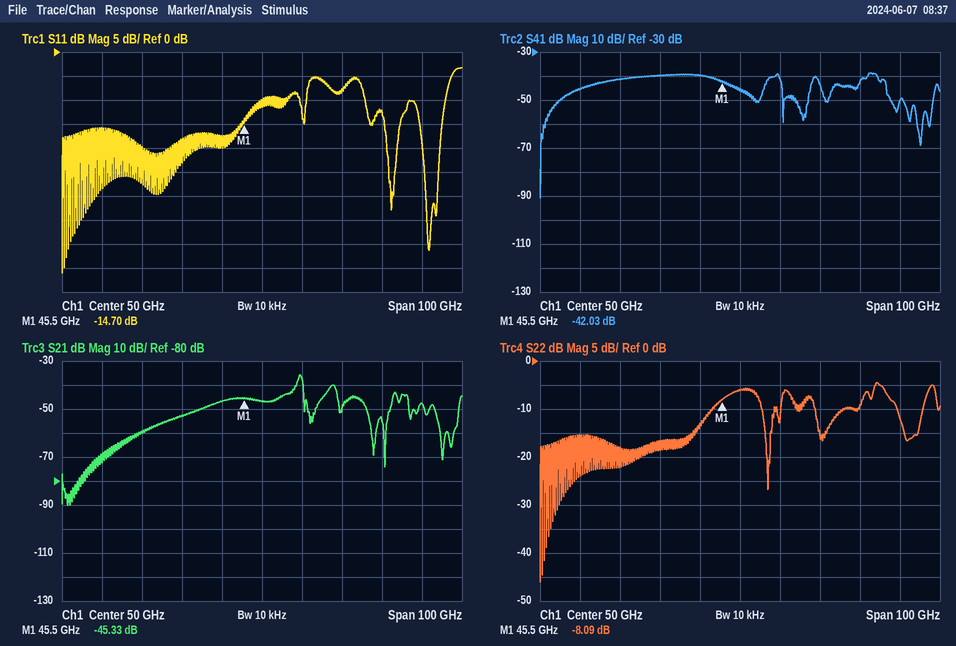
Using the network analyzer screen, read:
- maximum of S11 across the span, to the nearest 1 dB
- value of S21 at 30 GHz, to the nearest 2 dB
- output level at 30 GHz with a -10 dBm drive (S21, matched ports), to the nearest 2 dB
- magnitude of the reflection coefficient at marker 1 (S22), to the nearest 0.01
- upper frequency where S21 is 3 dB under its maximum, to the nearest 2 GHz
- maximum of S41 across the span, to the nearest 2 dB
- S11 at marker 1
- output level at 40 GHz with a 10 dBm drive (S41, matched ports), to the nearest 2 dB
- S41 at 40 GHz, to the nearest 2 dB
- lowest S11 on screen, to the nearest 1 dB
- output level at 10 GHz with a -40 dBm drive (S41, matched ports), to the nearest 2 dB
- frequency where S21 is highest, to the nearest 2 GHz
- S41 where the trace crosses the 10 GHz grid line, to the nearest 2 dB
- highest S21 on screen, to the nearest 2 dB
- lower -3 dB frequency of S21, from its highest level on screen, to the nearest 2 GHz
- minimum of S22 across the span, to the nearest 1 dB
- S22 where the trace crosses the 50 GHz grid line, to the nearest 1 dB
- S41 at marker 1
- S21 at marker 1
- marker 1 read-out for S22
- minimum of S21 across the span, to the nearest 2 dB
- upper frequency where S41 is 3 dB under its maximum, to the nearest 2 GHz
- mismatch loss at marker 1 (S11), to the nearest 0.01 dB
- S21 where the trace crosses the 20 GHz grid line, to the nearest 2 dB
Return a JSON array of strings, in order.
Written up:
["-3 dB", "-52 dB", "-62 dBm", "0.39", "60 GHz", "-38 dB", "-14.70 dB", "-30 dBm", "-40 dB", "-46 dB", "-86 dBm", "60 GHz", "-46 dB", "-36 dB", "58 GHz", "-46 dB", "-6 dB", "-42.03 dB", "-45.33 dB", "-8.09 dB", "-90 dB", "84 GHz", "0.15 dB", "-60 dB"]
